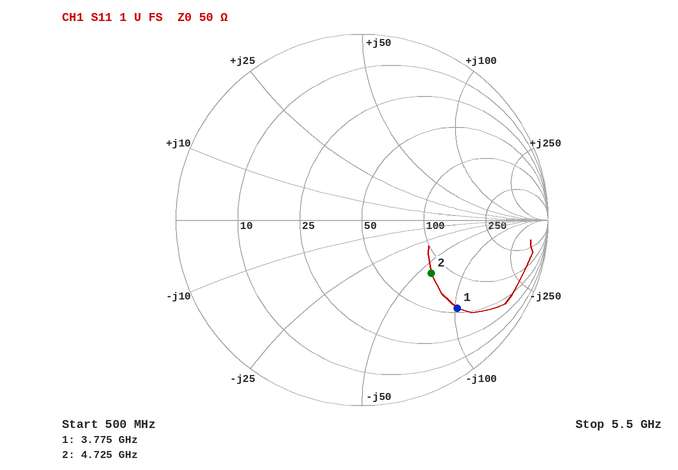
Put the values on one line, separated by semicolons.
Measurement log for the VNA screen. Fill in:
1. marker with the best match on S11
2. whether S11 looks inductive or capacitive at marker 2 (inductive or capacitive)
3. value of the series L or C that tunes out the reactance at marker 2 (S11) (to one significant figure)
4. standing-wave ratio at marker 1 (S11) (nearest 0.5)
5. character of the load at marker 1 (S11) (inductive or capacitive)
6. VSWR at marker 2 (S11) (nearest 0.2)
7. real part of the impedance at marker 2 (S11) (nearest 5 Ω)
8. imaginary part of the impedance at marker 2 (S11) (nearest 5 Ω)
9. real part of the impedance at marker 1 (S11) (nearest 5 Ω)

marker 2; capacitive; 2 nH; 5.5; capacitive; 2.8; 80 Ω; -60 Ω; 55 Ω
